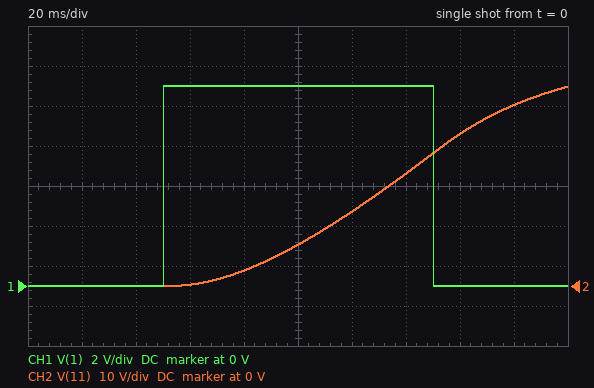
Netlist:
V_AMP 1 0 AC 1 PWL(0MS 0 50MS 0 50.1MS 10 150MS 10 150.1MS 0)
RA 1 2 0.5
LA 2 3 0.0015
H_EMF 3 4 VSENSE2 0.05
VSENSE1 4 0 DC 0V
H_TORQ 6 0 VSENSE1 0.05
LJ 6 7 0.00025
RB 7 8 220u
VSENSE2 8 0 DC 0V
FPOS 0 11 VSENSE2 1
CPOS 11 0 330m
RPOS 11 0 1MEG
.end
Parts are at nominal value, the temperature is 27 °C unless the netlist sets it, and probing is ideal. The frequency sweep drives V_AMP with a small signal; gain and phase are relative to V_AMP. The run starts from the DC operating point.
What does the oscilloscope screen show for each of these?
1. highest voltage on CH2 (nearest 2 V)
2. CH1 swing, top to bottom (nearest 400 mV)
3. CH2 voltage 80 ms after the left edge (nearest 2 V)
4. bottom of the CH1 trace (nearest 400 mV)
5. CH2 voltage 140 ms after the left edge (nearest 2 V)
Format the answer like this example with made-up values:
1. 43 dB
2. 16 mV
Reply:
1. 50 V
2. 10.0 V
3. 4 V
4. 0 V
5. 28 V
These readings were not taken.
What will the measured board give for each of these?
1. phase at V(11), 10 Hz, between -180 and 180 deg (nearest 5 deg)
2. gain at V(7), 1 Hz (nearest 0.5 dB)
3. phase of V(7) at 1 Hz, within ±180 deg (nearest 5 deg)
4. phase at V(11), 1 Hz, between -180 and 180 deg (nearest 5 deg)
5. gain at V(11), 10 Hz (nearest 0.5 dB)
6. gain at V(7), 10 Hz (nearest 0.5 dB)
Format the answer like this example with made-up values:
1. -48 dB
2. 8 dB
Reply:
1. -170 deg
2. -48.0 dB
3. -15 deg
4. -105 deg
5. -10.5 dB
6. -57.0 dB
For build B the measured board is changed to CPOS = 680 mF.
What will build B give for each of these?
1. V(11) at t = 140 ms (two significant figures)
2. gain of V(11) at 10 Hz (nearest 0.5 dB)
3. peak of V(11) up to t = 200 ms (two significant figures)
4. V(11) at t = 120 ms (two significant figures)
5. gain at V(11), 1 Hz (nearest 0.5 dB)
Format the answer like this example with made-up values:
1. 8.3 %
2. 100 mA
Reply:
1. 14 V
2. -16.5 dB
3. 24 V
4. 9.0 V
5. 12.5 dB
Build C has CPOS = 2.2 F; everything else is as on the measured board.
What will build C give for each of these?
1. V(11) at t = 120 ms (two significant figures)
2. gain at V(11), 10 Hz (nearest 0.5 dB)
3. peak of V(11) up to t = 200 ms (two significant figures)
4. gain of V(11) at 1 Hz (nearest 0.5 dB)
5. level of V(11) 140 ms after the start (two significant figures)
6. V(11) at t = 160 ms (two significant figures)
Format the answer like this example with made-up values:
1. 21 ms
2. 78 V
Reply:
1. 2.8 V
2. -27.0 dB
3. 7.5 V
4. 2.5 dB
5. 4.2 V
6. 5.7 V
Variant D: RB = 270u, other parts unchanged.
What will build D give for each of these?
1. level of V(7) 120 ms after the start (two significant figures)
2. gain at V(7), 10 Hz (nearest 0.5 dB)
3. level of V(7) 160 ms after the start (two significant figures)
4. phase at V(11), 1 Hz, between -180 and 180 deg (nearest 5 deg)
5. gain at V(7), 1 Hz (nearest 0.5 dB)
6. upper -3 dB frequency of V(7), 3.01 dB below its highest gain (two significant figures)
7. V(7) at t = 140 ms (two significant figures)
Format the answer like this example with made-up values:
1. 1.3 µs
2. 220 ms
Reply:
1. 40 mV
2. -55.5 dB
3. 39 mV
4. -105 deg
5. -46.0 dB
6. 3.6 Hz
7. 44 mV
